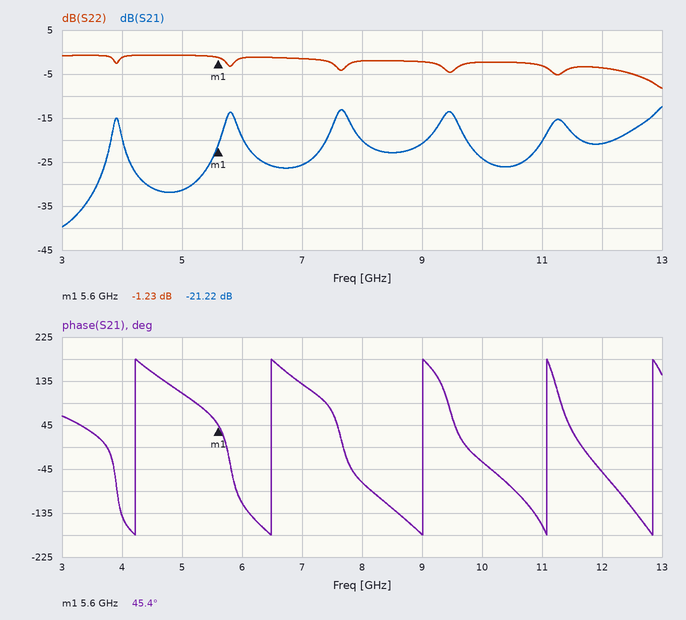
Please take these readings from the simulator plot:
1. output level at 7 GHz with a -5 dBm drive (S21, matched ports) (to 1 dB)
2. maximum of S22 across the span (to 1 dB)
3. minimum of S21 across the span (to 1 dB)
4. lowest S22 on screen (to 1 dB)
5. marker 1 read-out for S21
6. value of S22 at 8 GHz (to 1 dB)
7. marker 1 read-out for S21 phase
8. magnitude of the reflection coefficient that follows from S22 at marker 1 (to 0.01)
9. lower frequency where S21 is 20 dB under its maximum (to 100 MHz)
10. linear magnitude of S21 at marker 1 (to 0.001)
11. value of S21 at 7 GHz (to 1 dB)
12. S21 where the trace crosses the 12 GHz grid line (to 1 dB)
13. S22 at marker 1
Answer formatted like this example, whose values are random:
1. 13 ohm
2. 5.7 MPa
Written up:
1. -31 dBm
2. -1 dB
3. -40 dB
4. -8 dB
5. -21.22 dB
6. -2 dB
7. 45.4°
8. 0.87
9. 3.5 GHz
10. 0.087
11. -26 dB
12. -21 dB
13. -1.23 dB
